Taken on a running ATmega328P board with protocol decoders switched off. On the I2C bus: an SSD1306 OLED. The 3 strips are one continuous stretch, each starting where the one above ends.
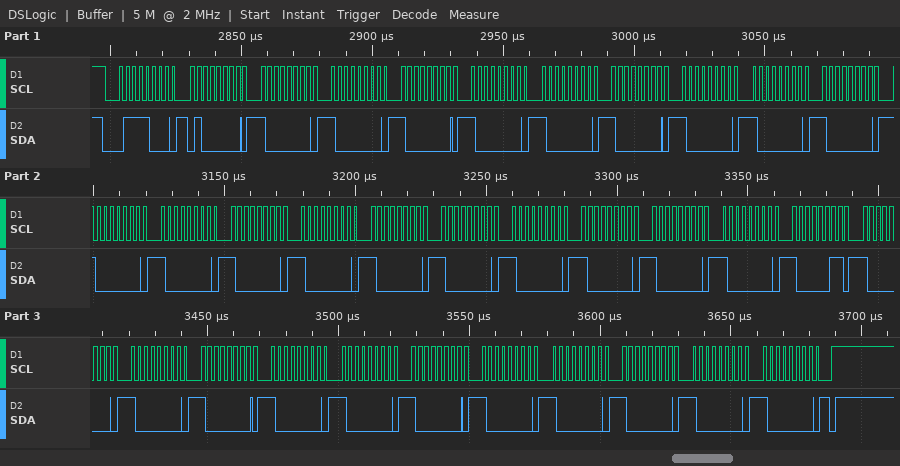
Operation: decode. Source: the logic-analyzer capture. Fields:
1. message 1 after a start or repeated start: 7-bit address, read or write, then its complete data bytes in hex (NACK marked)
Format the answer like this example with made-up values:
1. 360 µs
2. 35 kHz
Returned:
1. 0x3C write: 40 80 80 80 80 80 80 80 80 80 80 80 80 80 80 80 80 80 80 80 83 80 80 80 80 80 80 80 80 80 80 80
